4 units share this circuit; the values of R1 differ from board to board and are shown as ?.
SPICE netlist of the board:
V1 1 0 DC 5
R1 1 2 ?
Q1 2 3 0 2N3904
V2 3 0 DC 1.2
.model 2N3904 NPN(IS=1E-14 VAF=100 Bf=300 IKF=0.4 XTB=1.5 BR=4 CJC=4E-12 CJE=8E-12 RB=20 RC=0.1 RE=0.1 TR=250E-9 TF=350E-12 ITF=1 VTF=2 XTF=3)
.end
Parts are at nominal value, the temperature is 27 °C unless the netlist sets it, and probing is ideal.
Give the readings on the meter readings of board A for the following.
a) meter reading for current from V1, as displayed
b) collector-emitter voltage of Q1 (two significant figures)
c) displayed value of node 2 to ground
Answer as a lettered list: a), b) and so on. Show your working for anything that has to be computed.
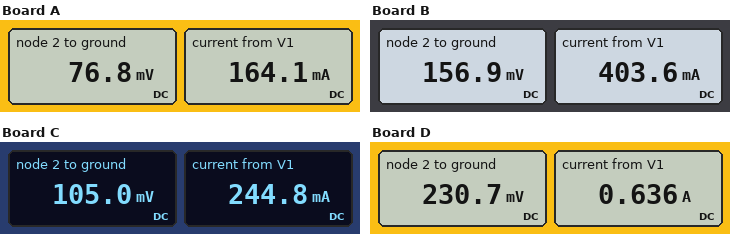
a) 164.1 mA
b) 76.8 mV = 77 mV
c) 76.8 mV
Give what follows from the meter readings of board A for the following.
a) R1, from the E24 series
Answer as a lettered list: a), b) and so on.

a) 30 Ω
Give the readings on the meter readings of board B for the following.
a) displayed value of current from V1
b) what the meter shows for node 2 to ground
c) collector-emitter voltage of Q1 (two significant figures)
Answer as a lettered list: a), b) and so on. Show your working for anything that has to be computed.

a) 403.6 mA
b) 156.9 mV
c) 156.9 mV = 160 mV
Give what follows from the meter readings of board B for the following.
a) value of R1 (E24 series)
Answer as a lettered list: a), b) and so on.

a) 12 Ω
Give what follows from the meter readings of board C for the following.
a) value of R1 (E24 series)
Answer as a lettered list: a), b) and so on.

a) 20 Ω
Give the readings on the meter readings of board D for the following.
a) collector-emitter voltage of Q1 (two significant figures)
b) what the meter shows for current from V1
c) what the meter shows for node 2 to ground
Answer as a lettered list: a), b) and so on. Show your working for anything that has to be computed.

a) 230.7 mV = 230 mV
b) 0.636 A
c) 230.7 mV
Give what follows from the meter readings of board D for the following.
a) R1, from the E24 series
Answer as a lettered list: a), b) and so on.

a) 7.5 Ω
